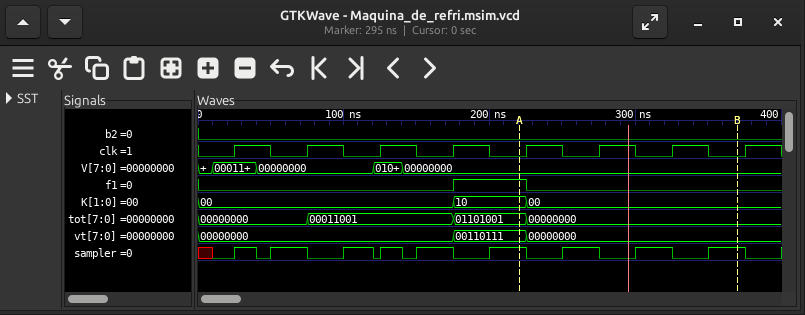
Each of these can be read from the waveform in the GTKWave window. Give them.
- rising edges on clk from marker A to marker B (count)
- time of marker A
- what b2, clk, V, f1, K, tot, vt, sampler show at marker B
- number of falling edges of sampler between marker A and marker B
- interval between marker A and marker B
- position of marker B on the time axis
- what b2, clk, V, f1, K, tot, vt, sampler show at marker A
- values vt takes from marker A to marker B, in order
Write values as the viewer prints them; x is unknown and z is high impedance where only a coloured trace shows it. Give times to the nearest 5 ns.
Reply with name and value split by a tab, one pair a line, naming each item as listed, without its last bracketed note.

rising edges on clk from marker A to marker B	3
time of marker A	220 ns
what b2, clk, V, f1, K, tot, vt, sampler show at marker B	b2=0, clk=0, V=00000000, f1=0, K=00, tot=00000000, vt=00000000, sampler=1
number of falling edges of sampler between marker A and marker B	3
interval between marker A and marker B	150 ns
position of marker B on the time axis	370 ns
what b2, clk, V, f1, K, tot, vt, sampler show at marker A	b2=0, clk=0, V=00000000, f1=1, K=10, tot=01101001, vt=00110111, sampler=1
values vt takes from marker A to marker B, in order	00110111, 00000000
